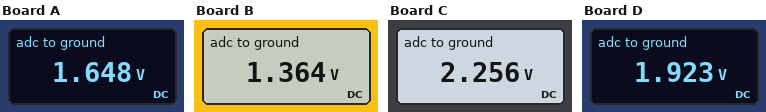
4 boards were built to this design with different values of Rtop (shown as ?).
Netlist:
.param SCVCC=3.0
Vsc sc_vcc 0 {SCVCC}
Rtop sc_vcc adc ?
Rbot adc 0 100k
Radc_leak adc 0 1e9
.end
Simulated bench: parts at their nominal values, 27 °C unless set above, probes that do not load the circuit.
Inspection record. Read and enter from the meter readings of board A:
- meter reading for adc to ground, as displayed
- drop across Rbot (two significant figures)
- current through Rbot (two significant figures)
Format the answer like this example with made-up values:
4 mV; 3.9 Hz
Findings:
1.648 V; 1.6 V; 16 µA
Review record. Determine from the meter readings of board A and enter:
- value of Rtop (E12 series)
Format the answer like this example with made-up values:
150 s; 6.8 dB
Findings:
82 kΩ
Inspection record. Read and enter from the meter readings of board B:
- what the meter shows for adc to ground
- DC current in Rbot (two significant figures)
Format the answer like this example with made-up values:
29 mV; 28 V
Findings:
1.364 V; 14 µA
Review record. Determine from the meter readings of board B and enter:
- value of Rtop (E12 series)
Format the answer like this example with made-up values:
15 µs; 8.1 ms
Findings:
120 kΩ
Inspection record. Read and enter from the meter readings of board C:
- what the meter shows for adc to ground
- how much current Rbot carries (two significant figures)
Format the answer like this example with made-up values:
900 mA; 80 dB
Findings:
2.256 V; 23 µA
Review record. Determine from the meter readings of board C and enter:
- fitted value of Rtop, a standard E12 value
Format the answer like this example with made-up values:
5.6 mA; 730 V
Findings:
33 kΩ
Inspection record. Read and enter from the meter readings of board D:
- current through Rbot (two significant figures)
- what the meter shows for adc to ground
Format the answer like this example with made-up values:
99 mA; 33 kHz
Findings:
19 µA; 1.923 V
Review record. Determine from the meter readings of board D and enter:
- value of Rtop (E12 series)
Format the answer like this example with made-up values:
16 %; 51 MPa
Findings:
56 kΩ
